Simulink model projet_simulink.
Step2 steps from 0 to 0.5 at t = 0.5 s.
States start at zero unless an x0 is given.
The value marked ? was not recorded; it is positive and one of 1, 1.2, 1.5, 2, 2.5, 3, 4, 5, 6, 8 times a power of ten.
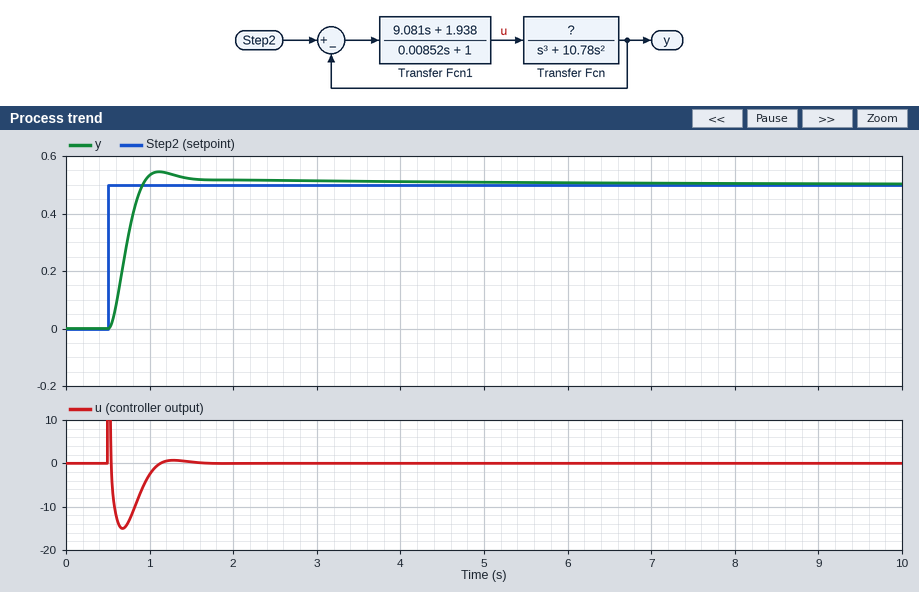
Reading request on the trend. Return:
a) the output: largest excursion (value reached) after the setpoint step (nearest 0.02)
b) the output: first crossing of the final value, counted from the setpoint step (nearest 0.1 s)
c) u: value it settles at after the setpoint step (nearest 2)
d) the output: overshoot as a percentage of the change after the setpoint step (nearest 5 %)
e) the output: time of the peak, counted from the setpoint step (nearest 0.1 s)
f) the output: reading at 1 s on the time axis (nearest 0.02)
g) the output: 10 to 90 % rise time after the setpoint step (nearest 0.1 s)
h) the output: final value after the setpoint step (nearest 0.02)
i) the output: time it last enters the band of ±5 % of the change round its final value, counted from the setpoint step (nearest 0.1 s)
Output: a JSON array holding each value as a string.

["0.54", "0.4 s", "0", "10 %", "0.6 s", "0.54", "0.3 s", "0.50", "0.9 s"]
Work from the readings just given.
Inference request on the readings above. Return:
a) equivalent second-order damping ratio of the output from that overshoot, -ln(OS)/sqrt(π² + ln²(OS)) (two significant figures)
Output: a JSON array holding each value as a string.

["0.59"]
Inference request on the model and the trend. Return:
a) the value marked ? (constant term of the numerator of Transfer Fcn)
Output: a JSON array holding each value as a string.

["6"]
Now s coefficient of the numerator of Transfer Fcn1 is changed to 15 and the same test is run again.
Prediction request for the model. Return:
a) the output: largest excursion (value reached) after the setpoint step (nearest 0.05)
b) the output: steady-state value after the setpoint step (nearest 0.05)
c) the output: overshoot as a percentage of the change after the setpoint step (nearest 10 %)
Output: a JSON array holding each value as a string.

["0.60", "0.50", "20 %"]
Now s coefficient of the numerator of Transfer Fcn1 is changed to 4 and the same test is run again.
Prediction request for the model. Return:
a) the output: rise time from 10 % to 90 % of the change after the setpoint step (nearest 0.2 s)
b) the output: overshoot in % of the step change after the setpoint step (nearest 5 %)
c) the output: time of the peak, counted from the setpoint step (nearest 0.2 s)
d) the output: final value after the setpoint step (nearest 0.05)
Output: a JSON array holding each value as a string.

["0.6 s", "15 %", "1.6 s", "0.50"]
